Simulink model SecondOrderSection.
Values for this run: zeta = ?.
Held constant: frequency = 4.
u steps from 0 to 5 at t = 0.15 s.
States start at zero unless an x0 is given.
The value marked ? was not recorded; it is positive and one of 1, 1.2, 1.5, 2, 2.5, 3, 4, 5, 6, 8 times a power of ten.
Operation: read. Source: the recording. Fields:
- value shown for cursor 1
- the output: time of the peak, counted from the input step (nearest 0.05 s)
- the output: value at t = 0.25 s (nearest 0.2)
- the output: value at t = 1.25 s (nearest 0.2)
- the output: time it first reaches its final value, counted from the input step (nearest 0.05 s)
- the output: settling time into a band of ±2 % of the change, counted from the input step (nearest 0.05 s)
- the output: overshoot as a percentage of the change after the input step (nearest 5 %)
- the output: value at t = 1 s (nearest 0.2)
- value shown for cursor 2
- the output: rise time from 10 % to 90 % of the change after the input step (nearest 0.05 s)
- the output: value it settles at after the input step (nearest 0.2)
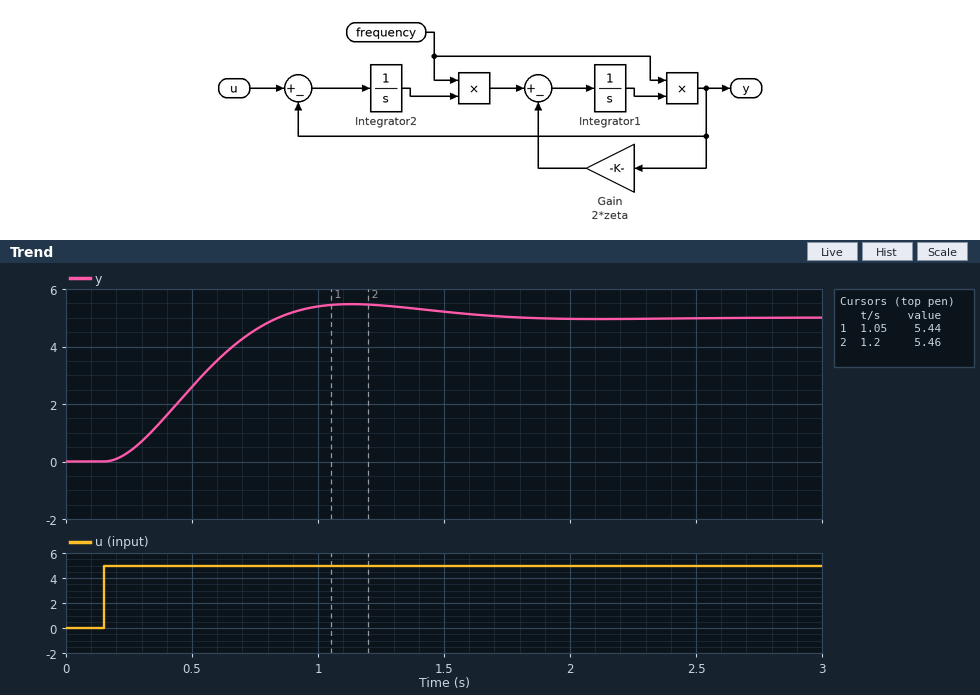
5.44
1.00 s
0.4
5.4
0.70 s
1.50 s
10 %
5.4
5.46
0.45 s
5.0
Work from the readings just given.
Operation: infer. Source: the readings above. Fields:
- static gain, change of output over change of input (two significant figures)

1.0
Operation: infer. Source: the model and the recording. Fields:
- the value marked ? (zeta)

0.6
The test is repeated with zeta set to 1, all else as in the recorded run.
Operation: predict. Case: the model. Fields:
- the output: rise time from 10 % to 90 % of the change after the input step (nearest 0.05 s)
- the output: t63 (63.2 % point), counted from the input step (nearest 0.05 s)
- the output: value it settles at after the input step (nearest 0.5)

0.85 s
0.55 s
5.0
